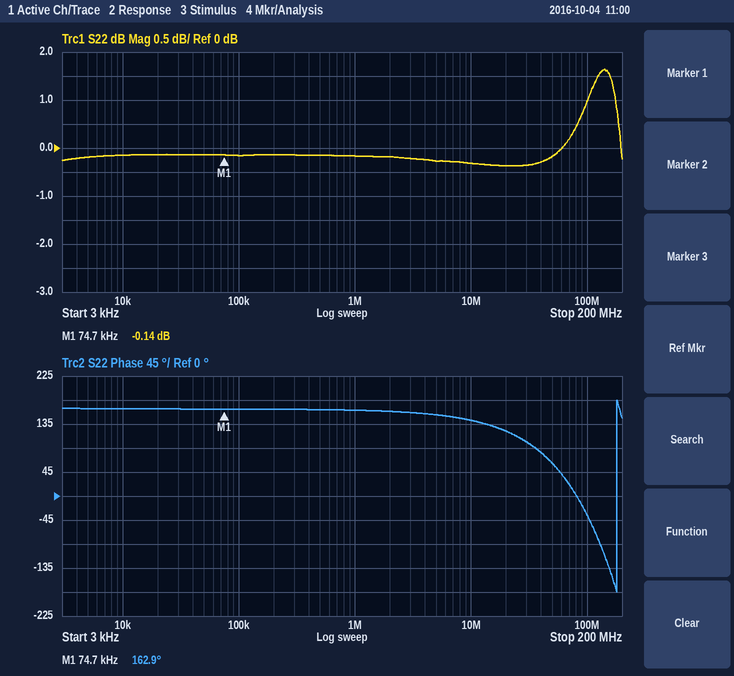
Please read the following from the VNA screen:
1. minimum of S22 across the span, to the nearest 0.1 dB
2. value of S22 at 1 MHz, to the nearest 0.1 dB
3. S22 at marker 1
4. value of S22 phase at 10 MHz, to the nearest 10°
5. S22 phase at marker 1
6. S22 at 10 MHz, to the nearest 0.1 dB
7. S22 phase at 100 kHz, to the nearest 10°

-0.4 dB
-0.2 dB
-0.14 dB
140°
162.9°
-0.3 dB
160°
